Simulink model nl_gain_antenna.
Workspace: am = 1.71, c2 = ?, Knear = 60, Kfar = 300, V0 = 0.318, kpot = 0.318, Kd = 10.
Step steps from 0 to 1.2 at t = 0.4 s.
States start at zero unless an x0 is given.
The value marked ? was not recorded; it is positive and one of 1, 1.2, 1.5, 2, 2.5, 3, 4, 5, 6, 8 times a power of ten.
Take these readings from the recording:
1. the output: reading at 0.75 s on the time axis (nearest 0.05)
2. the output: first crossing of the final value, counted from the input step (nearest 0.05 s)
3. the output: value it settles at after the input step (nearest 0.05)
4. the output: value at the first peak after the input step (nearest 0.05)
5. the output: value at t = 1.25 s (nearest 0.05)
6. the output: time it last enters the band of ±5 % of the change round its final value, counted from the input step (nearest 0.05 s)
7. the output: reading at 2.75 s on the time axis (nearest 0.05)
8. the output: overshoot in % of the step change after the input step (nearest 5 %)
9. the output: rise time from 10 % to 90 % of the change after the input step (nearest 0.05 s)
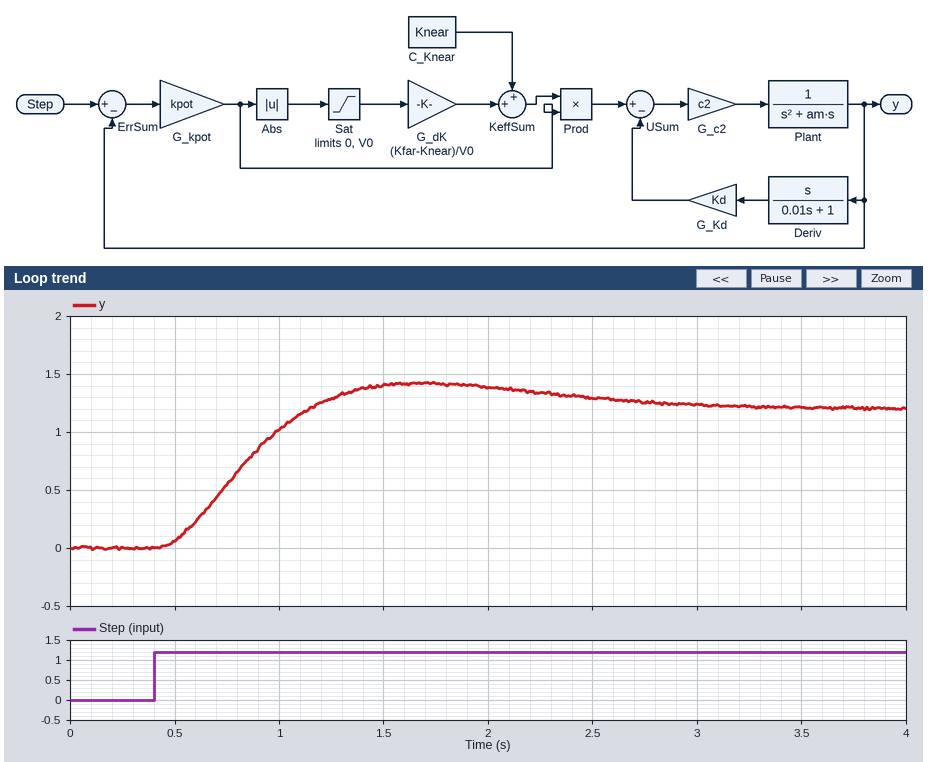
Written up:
0.55
0.75 s
1.20
1.40
1.30
2.35 s
1.25
20 %
0.50 s
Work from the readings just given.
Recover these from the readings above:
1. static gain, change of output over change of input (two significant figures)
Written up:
1.0
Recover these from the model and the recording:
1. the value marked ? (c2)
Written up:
0.12
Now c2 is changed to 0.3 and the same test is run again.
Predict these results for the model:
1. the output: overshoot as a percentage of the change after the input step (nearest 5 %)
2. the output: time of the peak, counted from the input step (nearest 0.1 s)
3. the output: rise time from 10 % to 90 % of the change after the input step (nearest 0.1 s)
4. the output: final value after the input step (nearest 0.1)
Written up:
15 %
0.8 s
0.3 s
1.2
